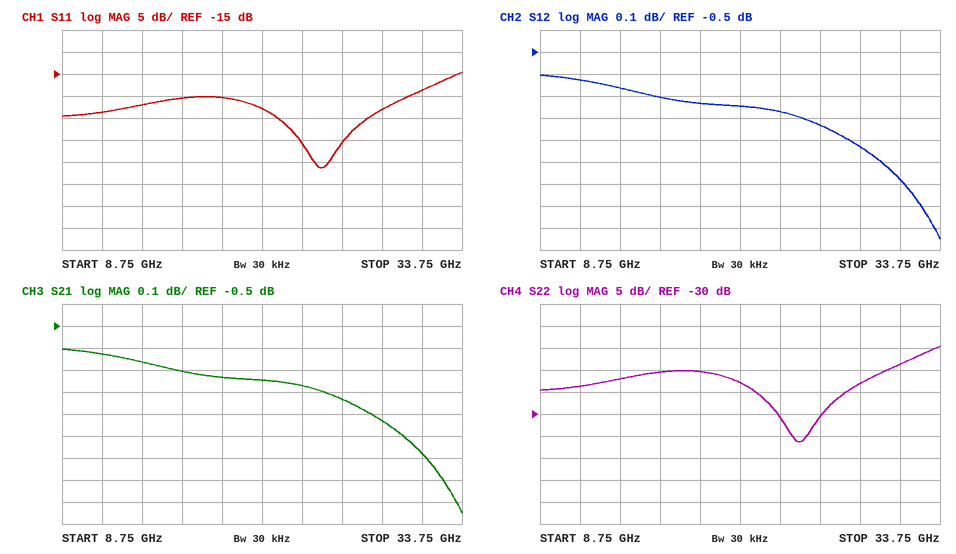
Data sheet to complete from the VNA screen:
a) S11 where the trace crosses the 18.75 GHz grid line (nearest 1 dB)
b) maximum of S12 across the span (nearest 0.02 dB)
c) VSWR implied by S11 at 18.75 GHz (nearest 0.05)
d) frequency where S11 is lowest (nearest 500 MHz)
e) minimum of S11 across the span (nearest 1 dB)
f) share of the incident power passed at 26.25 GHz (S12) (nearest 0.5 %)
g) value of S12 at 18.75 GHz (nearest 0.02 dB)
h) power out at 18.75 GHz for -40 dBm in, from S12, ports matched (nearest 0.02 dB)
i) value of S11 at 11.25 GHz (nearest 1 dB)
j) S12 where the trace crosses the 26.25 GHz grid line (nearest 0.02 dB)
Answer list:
-20 dB
-0.60 dB
1.20
25.0 GHz
-36 dB
82.5 %
-0.74 dB
-40.74 dBm
-24 dB
-0.84 dB
